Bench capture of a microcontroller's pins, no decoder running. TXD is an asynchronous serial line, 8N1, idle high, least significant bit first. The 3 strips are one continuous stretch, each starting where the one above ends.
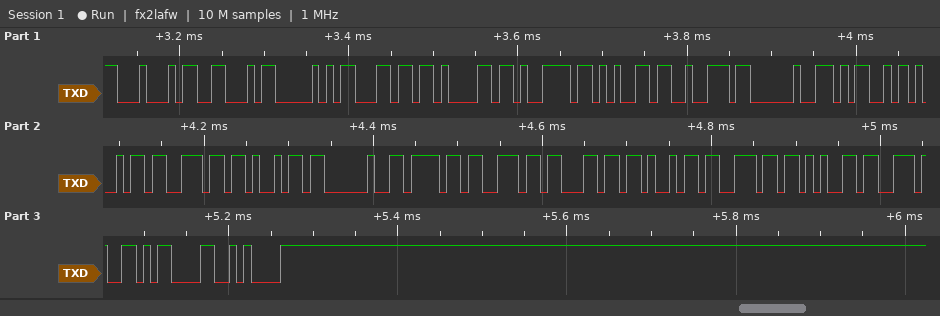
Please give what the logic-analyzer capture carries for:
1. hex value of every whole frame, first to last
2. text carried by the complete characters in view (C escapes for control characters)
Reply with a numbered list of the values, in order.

1. 44 46 50 6C 61 79 65 72 20 4D 69 6E 69 20 6F 6E 6C 69 6E 65 2E 0D 0A
2. "DFPlayer Mini online.\r\n"
